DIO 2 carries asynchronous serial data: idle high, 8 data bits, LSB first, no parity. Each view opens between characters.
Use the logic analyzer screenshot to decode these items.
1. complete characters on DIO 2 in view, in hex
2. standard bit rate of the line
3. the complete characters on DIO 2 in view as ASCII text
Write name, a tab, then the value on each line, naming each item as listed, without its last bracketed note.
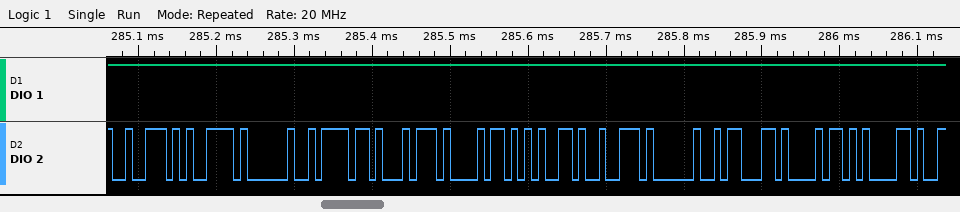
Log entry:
complete characters on DIO 2 in view, in hex	72, 79, 20, 6F, 74, 68, 65, 72, 20, 63, 68, 61
standard bit rate of the line	115200 baud
the complete characters on DIO 2 in view as ASCII text	"ry other cha"
